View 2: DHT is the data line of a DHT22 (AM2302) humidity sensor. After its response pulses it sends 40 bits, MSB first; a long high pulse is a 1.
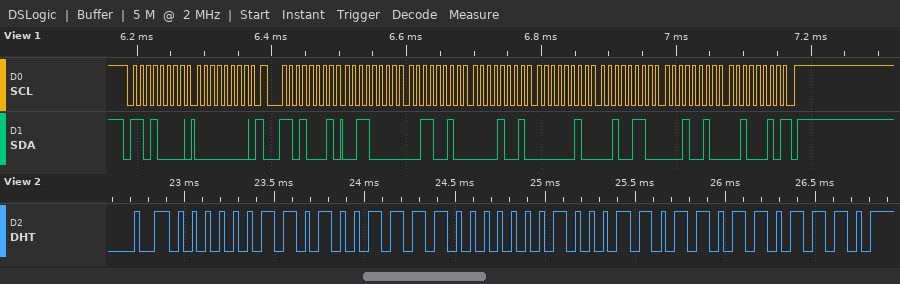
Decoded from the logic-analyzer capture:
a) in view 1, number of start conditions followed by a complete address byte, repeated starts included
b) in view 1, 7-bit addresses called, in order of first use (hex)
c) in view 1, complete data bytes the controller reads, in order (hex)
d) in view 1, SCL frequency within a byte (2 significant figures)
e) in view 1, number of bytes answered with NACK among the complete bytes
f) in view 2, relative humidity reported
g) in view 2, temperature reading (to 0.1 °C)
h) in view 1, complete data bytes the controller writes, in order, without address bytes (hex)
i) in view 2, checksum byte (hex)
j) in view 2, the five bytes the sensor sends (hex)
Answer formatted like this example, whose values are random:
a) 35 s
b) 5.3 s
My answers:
a) 2
b) 0x68
c) 30 32 09 02 26 12 22
d) 100 kHz
e) 1
f) 84.7 %
g) 28.3 °C
h) 00
i) 0x6E
j) 03 4F 01 1B 6E
